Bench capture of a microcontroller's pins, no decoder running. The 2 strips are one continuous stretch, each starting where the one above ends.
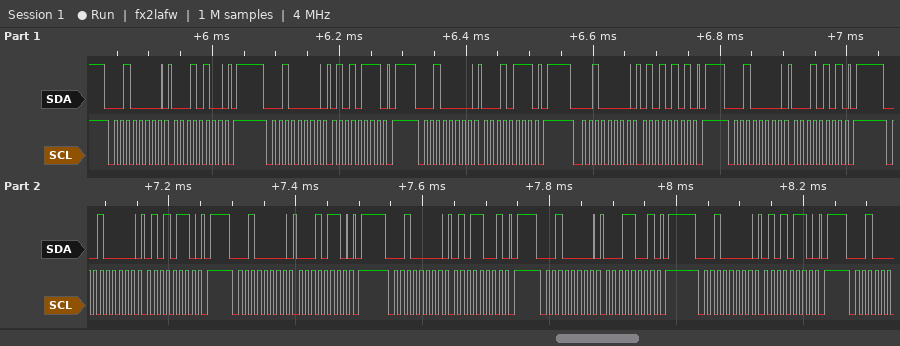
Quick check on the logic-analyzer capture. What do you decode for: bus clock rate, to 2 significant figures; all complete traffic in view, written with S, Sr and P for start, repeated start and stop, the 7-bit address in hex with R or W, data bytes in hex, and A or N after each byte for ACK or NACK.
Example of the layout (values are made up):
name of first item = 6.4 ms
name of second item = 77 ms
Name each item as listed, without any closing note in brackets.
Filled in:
bus clock rate, to 2 significant figures = 100 kHz
all complete traffic in view, written with S, Sr and P for start, repeated start and stop, the 7-bit address in hex with R or W, data bytes in hex, and A or N after each byte for ACK or NACK = S 10W A 14 A P S 10W A 57 A P S 10W A 17 A P S 10W A 55 A P S 10W A 15 A P S 10W A 56 A P S 10W A 16 A P S 10W A 59 A P S 10W A 19 A P S 10W A 56 A P
